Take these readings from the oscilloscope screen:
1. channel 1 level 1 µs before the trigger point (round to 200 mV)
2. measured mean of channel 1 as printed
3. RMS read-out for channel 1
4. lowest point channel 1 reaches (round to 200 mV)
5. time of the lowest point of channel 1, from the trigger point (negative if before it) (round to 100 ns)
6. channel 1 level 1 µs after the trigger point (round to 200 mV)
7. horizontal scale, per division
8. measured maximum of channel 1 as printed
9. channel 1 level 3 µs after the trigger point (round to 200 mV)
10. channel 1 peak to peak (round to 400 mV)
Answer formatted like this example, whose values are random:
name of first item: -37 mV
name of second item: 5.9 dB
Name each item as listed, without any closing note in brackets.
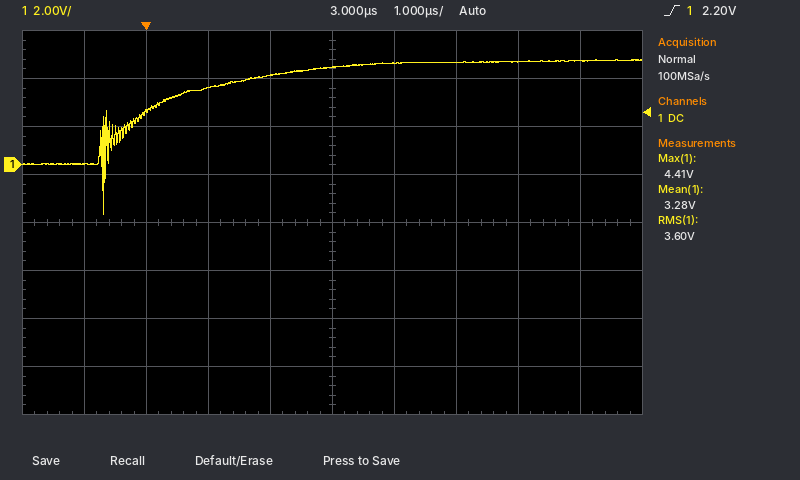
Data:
channel 1 level 1 µs before the trigger point: 0.0 V
measured mean of channel 1 as printed: 3.28 V
RMS read-out for channel 1: 3.60 V
lowest point channel 1 reaches: -2.0 V
time of the lowest point of channel 1, from the trigger point (negative if before it): -700 ns
channel 1 level 1 µs after the trigger point: 3.2 V
horizontal scale, per division: 1 µs
measured maximum of channel 1 as printed: 4.41 V
channel 1 level 3 µs after the trigger point: 4.0 V
channel 1 peak to peak: 6.4 V
